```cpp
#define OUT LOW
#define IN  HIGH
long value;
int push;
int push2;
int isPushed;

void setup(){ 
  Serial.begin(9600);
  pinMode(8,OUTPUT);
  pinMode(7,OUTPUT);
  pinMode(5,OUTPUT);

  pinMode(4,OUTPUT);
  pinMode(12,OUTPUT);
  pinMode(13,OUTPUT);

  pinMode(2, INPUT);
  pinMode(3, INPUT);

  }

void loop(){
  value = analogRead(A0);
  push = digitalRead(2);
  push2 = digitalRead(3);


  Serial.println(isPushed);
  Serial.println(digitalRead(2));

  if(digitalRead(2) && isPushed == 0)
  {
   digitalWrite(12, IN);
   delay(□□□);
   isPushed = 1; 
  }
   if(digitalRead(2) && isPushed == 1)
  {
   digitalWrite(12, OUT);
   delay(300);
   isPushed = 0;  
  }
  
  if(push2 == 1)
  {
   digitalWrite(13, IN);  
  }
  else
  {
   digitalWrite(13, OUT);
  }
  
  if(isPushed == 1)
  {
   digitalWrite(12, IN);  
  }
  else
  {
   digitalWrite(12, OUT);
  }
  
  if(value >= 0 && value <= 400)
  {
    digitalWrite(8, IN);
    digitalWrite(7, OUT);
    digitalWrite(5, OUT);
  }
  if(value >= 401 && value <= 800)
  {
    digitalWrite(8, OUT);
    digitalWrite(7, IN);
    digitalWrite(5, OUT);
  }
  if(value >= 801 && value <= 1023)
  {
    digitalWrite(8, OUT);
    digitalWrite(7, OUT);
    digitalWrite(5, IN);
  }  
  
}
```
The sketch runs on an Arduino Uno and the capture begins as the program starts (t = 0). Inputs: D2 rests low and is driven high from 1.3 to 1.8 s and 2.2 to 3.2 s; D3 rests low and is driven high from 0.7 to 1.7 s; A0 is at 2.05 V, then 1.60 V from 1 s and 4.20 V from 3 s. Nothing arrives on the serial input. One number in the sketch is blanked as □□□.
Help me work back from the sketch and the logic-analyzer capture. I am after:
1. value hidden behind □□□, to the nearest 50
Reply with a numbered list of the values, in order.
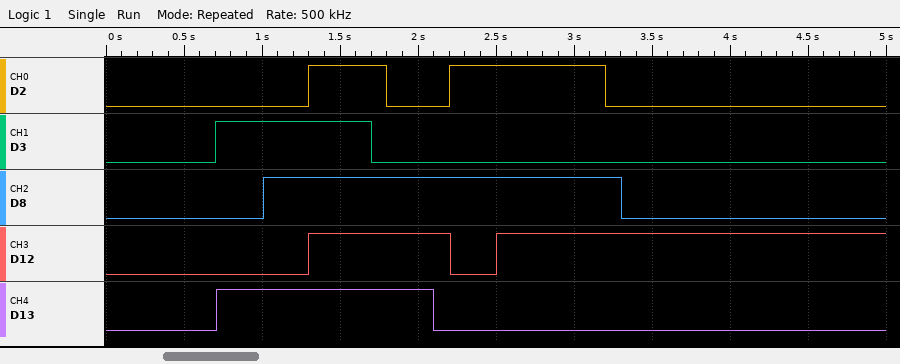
1. 800
